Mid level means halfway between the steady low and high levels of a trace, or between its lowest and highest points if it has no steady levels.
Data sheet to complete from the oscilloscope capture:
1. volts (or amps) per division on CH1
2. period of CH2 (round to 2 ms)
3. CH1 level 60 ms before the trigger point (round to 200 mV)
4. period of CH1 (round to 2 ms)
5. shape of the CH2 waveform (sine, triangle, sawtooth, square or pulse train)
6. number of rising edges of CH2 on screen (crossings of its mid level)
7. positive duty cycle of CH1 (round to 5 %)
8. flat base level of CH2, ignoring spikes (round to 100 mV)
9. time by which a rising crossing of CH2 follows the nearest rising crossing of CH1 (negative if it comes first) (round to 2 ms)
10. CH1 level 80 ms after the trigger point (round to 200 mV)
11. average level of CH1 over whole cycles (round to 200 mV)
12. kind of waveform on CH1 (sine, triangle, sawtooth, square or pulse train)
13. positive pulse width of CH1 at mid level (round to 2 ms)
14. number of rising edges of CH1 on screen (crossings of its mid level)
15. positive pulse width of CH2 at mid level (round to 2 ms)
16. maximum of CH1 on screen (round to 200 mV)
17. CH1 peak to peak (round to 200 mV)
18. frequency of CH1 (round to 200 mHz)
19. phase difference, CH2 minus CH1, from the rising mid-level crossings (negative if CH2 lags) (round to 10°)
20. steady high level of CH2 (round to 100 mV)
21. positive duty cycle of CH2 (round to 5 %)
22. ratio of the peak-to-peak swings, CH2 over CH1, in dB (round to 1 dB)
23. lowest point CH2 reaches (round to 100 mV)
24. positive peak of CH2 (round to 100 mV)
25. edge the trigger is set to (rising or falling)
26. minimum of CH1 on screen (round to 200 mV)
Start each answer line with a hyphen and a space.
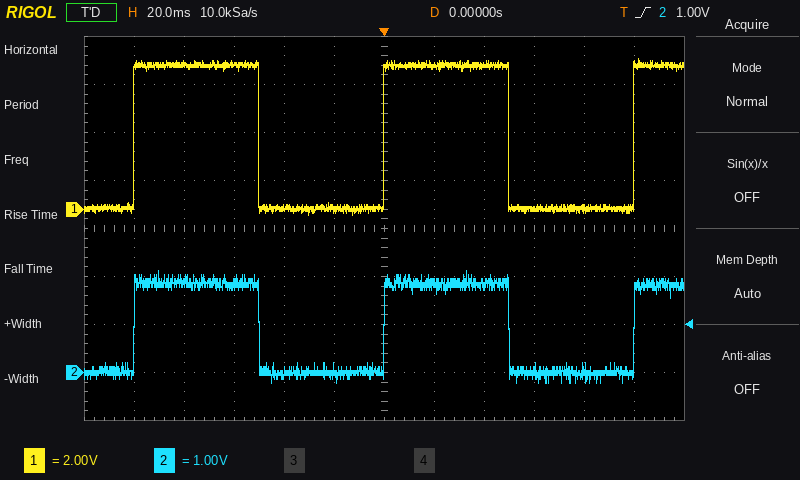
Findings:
- 2 V
- 100 ms
- 6.0 V
- 100 ms
- square
- 3
- 50 %
- 0.0 V
- 0 ms
- 0.0 V
- 3.0 V
- square
- 50 ms
- 3
- 50 ms
- 6.2 V
- 6.4 V
- 10.0 Hz
- 0°
- 1.9 V
- 50 %
- -9 dB
- -200 mV
- 2.1 V
- rising
- -200 mV
